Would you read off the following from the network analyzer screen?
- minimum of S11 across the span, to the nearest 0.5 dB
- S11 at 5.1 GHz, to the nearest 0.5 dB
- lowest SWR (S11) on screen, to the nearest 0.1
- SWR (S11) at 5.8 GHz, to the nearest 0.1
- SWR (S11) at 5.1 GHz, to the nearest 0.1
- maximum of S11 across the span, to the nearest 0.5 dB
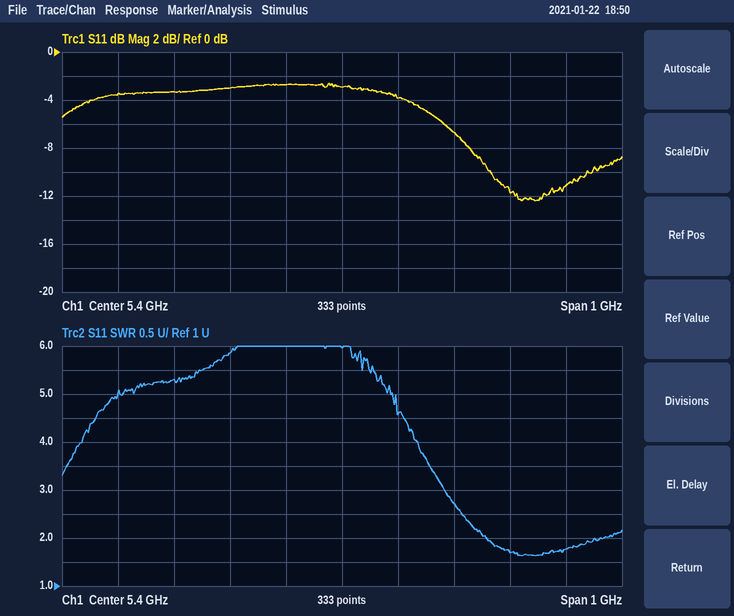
-12.5 dB
-3.5 dB
1.6
1.8
5.3
-2.5 dB
